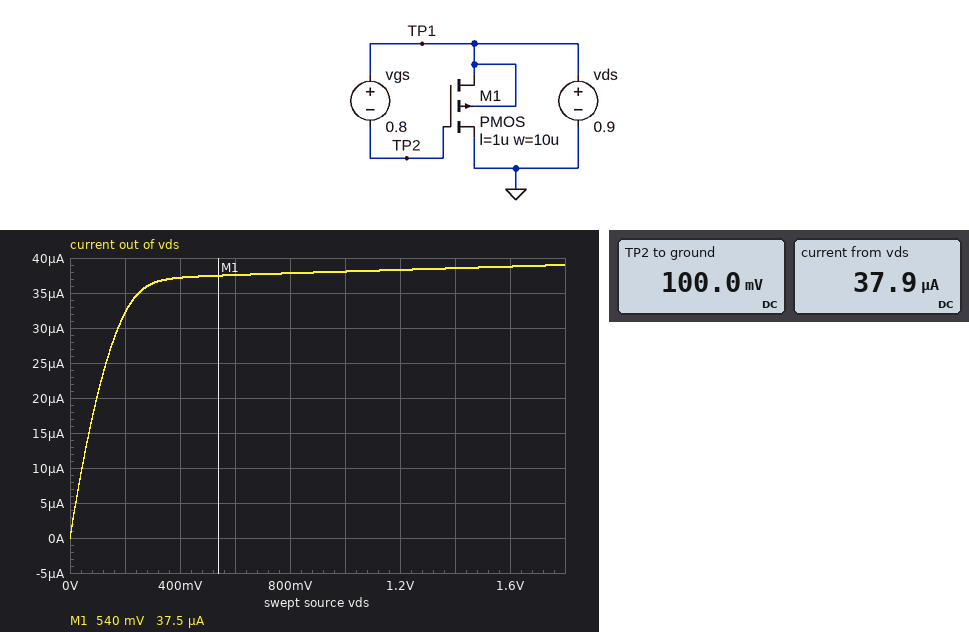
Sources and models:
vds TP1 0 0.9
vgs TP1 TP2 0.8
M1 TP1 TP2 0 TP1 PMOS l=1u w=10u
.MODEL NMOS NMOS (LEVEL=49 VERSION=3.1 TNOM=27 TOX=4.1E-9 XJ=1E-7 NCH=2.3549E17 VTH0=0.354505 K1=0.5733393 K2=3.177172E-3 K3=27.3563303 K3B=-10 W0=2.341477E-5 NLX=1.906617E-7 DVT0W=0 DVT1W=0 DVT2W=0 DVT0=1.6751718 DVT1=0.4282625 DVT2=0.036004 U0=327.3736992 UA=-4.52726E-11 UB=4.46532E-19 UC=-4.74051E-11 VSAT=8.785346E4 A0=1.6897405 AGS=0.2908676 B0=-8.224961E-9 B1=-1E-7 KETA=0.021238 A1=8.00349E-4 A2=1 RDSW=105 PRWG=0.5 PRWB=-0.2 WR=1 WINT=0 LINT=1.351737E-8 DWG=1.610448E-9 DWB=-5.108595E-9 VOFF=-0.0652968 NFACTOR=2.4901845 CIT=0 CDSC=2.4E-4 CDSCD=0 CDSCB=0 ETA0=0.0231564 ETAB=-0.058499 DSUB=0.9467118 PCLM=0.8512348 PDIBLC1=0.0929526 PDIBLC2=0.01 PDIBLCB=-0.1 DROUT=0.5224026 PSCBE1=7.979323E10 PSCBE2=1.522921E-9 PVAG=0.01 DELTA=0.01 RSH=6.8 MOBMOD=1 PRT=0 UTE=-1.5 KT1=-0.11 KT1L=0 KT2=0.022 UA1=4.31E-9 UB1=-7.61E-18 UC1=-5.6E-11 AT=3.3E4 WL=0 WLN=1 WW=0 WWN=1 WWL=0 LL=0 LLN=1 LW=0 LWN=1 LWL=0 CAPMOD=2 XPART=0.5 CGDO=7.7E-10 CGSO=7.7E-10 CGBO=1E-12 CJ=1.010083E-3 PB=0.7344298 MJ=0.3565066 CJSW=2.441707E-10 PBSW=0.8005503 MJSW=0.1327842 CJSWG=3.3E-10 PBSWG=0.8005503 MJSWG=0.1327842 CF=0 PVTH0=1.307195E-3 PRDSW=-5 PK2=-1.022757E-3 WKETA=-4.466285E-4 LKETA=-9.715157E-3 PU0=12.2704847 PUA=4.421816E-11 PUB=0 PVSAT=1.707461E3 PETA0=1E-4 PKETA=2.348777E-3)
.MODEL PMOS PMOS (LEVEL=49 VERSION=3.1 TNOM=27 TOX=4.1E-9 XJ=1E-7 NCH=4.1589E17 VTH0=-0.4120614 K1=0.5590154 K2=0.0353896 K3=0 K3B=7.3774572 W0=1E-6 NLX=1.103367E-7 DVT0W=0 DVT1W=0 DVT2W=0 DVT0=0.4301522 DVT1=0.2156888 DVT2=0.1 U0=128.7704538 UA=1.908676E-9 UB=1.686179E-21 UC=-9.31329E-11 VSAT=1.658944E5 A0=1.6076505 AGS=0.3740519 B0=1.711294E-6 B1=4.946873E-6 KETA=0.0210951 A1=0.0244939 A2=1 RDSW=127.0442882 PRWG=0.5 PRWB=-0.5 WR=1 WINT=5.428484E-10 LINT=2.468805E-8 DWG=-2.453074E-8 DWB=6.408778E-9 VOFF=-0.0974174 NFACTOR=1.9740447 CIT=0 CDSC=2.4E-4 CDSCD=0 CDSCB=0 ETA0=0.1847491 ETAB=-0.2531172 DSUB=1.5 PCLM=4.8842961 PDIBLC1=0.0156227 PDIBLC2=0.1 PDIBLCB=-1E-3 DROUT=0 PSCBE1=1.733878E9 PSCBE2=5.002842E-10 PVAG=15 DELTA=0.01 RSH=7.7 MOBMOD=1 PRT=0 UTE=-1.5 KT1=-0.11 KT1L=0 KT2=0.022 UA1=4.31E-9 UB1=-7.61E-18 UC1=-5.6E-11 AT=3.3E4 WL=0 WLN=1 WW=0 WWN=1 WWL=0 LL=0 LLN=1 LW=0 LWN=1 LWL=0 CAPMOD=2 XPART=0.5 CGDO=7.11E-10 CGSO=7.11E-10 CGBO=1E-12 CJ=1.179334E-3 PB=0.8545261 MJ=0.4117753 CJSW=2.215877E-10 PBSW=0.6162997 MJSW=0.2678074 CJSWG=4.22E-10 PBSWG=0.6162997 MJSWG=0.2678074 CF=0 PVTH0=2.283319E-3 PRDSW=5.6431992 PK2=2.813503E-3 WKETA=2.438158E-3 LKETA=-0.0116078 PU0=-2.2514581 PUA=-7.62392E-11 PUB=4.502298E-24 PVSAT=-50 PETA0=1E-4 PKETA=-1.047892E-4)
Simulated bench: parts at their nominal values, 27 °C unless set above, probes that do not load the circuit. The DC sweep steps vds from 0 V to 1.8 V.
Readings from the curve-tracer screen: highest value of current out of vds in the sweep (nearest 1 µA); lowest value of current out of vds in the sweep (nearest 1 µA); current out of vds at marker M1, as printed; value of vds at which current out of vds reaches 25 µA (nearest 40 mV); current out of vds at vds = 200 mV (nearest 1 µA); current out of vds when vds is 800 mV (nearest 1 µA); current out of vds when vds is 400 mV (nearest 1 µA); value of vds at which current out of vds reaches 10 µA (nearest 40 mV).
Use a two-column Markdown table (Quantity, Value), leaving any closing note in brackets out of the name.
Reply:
| Quantity | Value |
|---|---|
| highest value of current out of vds in the sweep | 39 µA |
| lowest value of current out of vds in the sweep | 0 A |
| current out of vds at marker M1, as printed | 37.5 µA |
| value of vds at which current out of vds reaches 25 µA | 120 mV |
| current out of vds at vds = 200 mV | 32 µA |
| current out of vds when vds is 800 mV | 38 µA |
| current out of vds when vds is 400 mV | 37 µA |
| value of vds at which current out of vds reaches 10 µA | 40 mV |
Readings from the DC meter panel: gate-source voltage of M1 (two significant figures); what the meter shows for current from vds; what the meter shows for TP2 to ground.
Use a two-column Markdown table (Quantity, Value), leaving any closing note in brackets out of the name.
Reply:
| Quantity | Value |
|---|---|
| gate-source voltage of M1 | 100 mV |
| what the meter shows for current from vds | 37.9 µA |
| what the meter shows for TP2 to ground | 100.0 mV |
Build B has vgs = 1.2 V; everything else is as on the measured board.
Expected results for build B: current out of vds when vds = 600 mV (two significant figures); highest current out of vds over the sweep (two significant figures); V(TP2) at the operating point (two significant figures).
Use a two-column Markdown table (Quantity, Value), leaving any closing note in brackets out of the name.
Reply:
| Quantity | Value |
|---|---|
| current out of vds when vds = 600 mV | 140 µA |
| highest current out of vds over the sweep | 150 µA |
| V(TP2) at the operating point | -300 mV |
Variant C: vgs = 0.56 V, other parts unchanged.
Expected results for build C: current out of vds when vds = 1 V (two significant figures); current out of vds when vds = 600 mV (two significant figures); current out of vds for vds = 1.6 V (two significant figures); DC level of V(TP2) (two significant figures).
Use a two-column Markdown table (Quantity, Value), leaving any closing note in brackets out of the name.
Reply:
| Quantity | Value |
|---|---|
| current out of vds when vds = 1 V | 5.1 µA |
| current out of vds when vds = 600 mV | 5.0 µA |
| current out of vds for vds = 1.6 V | 5.2 µA |
| DC level of V(TP2) | 340 mV |
